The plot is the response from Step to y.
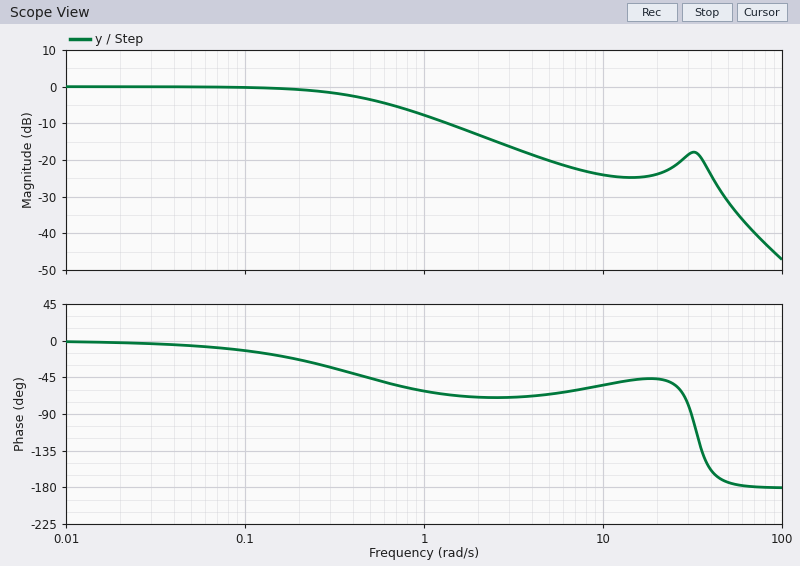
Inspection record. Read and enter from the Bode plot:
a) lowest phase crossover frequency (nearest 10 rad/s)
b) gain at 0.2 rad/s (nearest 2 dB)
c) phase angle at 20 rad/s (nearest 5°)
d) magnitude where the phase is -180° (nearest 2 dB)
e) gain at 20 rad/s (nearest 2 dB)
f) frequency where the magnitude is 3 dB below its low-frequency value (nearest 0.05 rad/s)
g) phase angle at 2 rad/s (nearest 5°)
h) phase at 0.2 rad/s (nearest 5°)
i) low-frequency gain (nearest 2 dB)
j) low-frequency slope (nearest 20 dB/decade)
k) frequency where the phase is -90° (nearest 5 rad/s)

80 rad/s
0 dB
-45°
-42 dB
-24 dB
0.45 rad/s
-70°
-25°
0 dB
0 dB/decade
30 rad/s
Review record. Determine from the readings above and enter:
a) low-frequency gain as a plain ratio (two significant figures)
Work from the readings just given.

1.0
